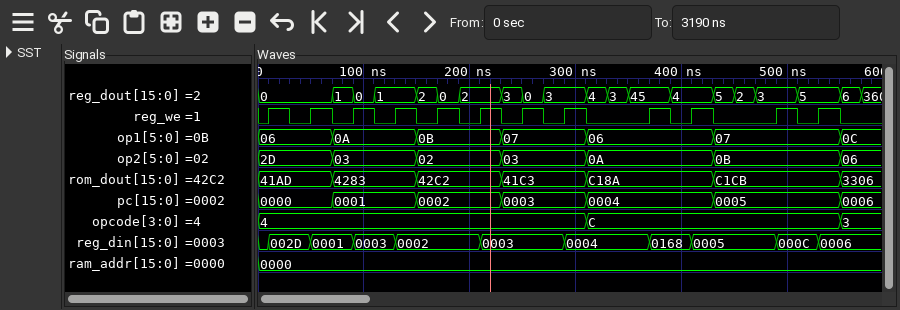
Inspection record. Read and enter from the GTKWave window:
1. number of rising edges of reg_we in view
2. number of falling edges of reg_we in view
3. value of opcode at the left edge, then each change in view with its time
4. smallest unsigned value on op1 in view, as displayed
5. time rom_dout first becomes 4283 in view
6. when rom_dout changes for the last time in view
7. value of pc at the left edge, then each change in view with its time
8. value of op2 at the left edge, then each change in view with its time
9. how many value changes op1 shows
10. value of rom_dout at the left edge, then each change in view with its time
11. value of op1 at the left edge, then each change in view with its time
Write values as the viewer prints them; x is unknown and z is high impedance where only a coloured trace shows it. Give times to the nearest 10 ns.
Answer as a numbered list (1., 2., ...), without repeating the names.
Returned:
1. 12
2. 12
3. 4, C at 310 ns, 3 at 550 ns
4. 06
5. 70 ns
6. 550 ns
7. 0000, 0001 at 70 ns, 0002 at 150 ns, 0003 at 230 ns, 0004 at 310 ns, 0005 at 430 ns, 0006 at 550 ns
8. 2D, 03 at 70 ns, 02 at 150 ns, 03 at 230 ns, 0A at 310 ns, 0B at 430 ns, 06 at 550 ns
9. 6
10. 41AD, 4283 at 70 ns, 42C2 at 150 ns, 41C3 at 230 ns, C18A at 310 ns, C1CB at 430 ns, 3306 at 550 ns
11. 06, 0A at 70 ns, 0B at 150 ns, 07 at 230 ns, 06 at 310 ns, 07 at 430 ns, 0C at 550 ns
